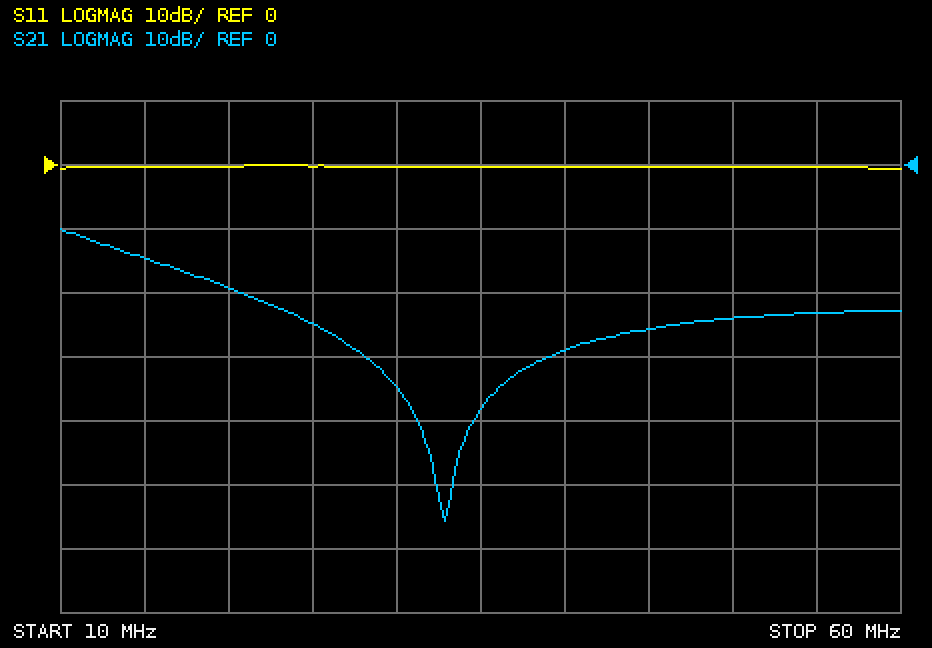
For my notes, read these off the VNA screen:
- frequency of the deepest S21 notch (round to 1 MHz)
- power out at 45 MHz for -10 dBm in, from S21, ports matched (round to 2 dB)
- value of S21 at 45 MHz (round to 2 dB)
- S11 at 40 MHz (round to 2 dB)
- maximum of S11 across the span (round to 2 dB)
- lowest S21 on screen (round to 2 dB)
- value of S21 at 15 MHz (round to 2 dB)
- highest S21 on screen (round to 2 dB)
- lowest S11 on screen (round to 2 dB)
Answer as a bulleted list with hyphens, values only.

- 33 MHz
- -36 dBm
- -26 dB
- 0 dB
- 0 dB
- -56 dB
- -14 dB
- -10 dB
- 0 dB
